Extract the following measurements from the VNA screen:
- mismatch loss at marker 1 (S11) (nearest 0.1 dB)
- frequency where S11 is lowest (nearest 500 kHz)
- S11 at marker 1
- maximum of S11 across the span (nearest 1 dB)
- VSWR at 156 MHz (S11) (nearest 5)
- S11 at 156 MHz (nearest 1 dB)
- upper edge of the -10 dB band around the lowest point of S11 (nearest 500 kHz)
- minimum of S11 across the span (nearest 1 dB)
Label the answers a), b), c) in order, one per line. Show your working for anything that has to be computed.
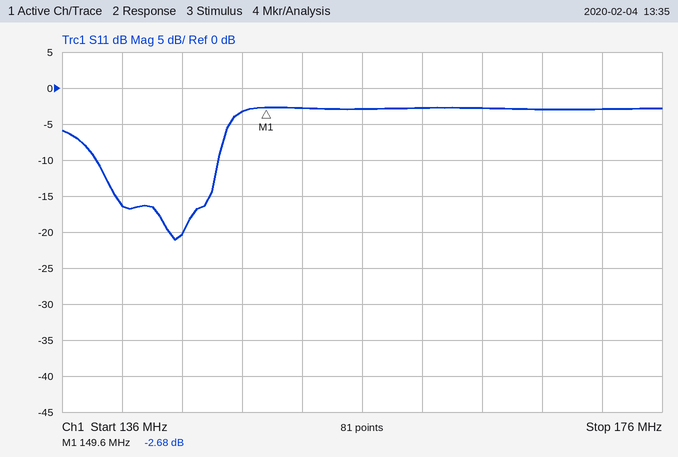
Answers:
a) −10 log10(1 − 10^(-2.68/10)) ≈ 3.4 dB
b) 143.5 MHz
c) -2.68 dB
d) -3 dB
e) |Γ| = 10^(-3/20) = 0.7079; VSWR = (1 + 0.7079)/(1 − 0.7079) ≈ 5.85, so 5 to the nearest 5
f) -3 dB
g) 146.5 MHz
h) -21 dB
